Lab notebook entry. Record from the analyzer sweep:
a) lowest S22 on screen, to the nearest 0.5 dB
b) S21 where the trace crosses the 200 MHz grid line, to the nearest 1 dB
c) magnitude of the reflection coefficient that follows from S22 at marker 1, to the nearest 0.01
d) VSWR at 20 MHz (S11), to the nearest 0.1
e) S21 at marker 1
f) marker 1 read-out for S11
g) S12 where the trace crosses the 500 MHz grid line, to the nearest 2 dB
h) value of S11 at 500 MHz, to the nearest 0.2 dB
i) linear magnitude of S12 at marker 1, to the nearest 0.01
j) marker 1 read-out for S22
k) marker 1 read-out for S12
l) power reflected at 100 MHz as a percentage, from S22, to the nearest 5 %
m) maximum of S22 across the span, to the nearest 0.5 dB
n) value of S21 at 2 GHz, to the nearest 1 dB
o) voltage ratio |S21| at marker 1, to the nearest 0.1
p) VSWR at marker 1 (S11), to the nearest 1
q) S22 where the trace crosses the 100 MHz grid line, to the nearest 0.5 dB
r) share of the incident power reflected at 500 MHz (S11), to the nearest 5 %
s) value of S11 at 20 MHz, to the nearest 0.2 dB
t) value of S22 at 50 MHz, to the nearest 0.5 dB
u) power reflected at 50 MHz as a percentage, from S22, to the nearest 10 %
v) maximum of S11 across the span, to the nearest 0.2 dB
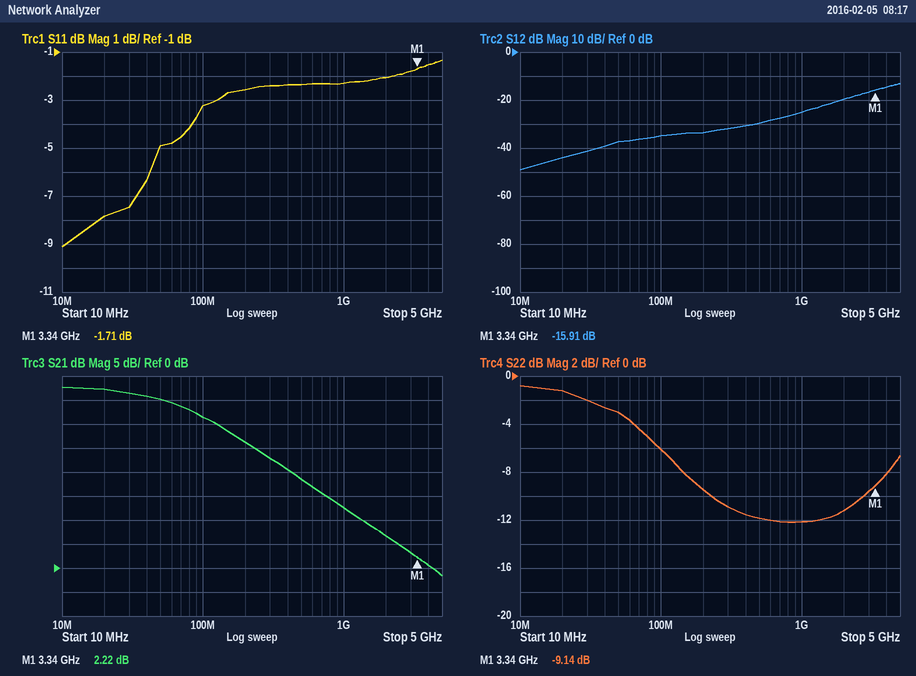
-12.0 dB
26 dB
0.35
2.4
2.22 dB
-1.71 dB
-30 dB
-2.4 dB
0.16
-9.14 dB
-15.91 dB
25 %
-1.0 dB
7 dB
1.3
10
-6.0 dB
60 %
-7.8 dB
-3.0 dB
50 %
-1.4 dB
